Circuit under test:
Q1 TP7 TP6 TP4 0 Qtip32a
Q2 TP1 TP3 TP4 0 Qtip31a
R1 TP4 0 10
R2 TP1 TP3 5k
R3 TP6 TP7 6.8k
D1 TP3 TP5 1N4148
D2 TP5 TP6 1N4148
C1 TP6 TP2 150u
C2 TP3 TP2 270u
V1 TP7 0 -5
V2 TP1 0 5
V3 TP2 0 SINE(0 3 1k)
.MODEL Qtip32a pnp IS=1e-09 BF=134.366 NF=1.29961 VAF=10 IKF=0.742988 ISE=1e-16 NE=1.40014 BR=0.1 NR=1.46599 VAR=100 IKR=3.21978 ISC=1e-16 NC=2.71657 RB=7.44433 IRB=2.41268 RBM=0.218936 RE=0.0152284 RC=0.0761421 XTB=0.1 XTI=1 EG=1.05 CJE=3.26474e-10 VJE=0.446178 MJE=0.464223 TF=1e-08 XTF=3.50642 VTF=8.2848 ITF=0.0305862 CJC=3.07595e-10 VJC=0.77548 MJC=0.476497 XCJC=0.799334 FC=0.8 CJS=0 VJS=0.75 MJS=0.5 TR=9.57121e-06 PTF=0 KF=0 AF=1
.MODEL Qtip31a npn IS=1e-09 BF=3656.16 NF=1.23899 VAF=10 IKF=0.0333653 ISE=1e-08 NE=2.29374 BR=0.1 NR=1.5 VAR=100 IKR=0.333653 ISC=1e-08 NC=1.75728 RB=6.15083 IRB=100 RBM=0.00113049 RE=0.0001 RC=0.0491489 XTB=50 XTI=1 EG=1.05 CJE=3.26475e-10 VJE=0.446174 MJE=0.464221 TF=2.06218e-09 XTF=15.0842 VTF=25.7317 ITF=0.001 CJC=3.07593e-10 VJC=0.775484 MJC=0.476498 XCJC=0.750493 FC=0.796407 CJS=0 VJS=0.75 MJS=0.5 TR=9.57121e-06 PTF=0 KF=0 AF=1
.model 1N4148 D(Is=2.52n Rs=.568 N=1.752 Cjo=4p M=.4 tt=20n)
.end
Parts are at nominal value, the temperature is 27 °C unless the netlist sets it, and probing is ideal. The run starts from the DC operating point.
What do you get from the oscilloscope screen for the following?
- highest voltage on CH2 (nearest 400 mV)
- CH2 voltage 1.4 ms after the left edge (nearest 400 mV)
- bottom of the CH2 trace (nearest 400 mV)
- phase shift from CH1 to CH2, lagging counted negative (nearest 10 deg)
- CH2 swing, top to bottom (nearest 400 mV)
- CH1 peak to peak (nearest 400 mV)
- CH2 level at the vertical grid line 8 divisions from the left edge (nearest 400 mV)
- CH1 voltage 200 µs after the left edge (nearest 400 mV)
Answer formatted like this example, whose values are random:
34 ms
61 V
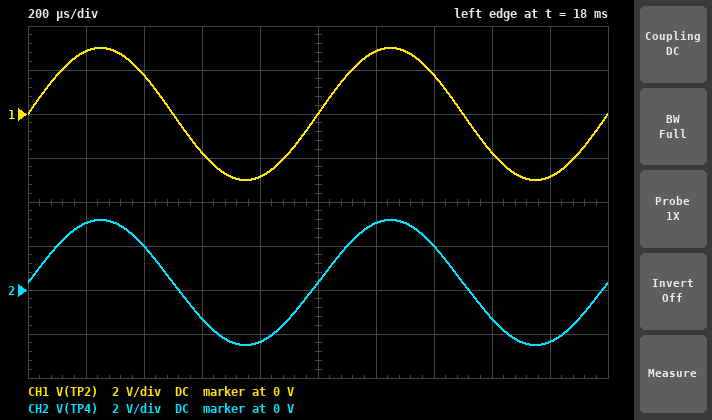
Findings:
3.2 V
2.0 V
-2.4 V
0 deg
5.6 V
6.0 V
-1.2 V
2.8 V
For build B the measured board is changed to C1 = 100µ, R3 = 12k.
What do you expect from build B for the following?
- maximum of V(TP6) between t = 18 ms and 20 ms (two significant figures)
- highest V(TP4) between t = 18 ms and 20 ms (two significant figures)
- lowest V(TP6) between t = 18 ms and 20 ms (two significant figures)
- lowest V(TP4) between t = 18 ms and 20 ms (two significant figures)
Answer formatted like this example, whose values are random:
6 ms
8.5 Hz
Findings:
3.3 V
3.6 V
-2.7 V
-2.0 V
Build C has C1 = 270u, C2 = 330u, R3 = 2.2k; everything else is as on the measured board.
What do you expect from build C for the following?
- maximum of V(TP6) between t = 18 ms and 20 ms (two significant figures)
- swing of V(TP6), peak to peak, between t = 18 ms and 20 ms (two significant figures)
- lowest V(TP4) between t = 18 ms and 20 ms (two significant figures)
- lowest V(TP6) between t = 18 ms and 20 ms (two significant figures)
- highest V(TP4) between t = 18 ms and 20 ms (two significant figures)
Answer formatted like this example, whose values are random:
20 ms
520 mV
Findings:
1.6 V
6.0 V
-3.7 V
-4.4 V
2.0 V
